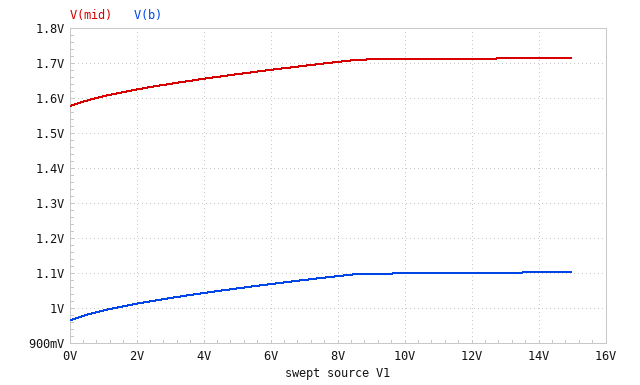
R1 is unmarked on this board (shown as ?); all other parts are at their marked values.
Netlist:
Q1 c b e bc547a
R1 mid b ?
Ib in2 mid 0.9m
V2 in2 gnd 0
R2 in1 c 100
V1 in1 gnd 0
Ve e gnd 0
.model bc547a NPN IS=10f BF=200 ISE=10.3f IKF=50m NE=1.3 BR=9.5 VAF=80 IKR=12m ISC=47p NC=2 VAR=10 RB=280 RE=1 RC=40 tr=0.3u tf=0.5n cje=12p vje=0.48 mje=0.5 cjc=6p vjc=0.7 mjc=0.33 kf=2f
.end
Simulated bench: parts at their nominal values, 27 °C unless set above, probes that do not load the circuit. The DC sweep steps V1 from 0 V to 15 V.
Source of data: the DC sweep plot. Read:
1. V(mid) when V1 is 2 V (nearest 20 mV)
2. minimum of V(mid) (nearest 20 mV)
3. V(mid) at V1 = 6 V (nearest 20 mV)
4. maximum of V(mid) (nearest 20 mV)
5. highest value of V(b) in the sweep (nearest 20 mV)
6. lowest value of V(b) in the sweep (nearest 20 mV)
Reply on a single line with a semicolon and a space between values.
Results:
1.62 V; 1.58 V; 1.68 V; 1.72 V; 1.10 V; 960 mV
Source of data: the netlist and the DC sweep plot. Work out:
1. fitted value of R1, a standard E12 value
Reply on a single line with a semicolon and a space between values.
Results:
680 Ω
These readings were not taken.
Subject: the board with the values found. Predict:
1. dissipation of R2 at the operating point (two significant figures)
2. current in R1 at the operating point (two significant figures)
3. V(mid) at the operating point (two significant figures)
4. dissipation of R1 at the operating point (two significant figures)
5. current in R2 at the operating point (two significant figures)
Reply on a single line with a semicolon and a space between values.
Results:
130 nW; 900 µA; 1.6 V; 550 µW; 36 µA
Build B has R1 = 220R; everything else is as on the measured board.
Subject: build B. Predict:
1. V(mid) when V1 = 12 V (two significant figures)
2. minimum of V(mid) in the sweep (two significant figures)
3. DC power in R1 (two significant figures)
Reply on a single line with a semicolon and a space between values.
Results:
1.3 V; 1.2 V; 180 µW
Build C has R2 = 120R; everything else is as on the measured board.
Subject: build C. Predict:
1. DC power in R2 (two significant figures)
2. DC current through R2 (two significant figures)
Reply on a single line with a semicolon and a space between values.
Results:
120 nW; 32 µA
